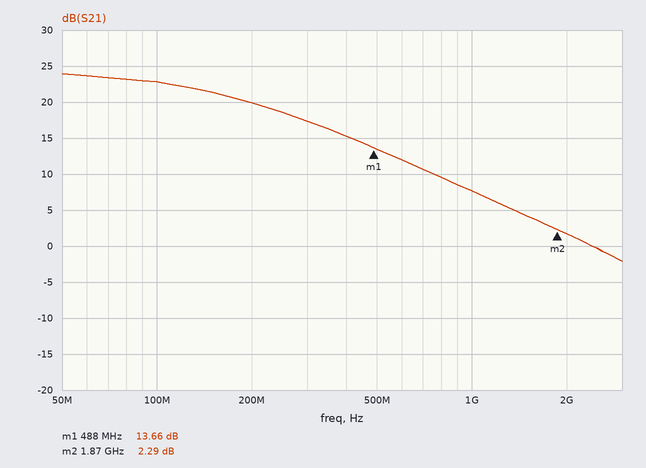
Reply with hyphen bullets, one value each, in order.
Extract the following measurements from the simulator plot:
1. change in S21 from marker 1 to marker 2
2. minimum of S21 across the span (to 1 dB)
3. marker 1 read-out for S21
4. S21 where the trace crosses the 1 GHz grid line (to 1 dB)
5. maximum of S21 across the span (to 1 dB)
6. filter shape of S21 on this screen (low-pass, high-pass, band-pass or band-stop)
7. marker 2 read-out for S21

- -11.37 dB
- -2 dB
- 13.66 dB
- 8 dB
- 24 dB
- low-pass
- 2.29 dB
